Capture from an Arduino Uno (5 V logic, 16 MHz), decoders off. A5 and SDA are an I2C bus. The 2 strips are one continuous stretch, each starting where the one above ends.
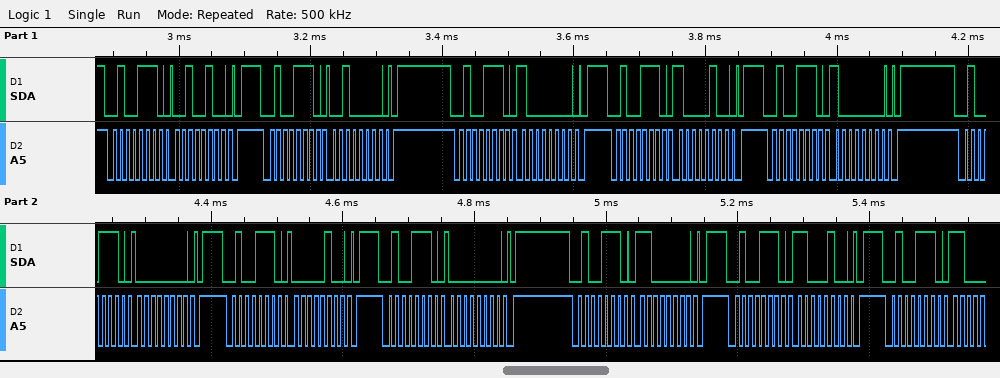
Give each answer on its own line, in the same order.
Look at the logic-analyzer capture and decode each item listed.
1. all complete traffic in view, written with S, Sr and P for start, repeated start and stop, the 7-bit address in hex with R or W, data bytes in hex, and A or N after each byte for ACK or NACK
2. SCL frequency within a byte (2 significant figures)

S 27W A 24 A P S 27W A 20 A P S 27W A 80 A P S 27W A 84 A P S 27W A 80 A P S 27W A 00 A P S 27W A 04 A P S 27W A 00 A P S 27W A C0 A P S 27W A C4 A P S 27W A
100 kHz
